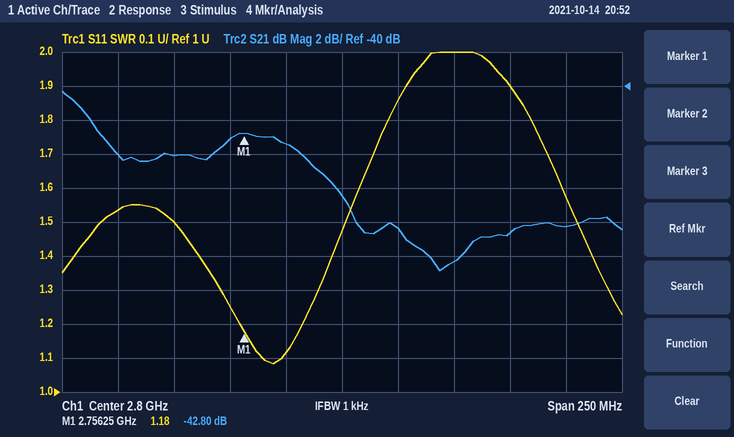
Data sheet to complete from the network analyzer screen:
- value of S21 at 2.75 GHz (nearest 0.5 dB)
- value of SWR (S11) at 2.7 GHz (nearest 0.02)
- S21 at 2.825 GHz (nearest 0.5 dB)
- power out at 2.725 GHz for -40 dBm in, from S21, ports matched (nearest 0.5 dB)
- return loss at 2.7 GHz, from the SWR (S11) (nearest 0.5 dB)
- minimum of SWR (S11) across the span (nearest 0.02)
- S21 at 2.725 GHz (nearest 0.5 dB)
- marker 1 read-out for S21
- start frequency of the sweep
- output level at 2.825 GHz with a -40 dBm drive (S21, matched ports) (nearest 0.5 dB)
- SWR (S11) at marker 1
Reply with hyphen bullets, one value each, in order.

- -43.0 dB
- 1.54
- -48.5 dB
- -84.0 dBm
- 13.5 dB
- 1.08
- -44.0 dB
- -42.80 dB
- 2.675 GHz
- -88.5 dBm
- 1.18
